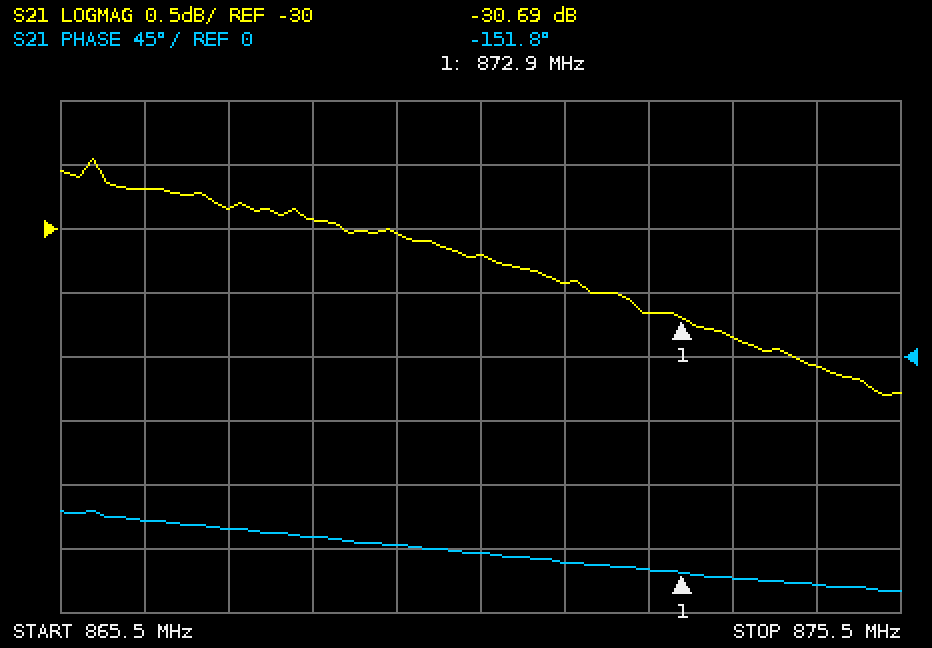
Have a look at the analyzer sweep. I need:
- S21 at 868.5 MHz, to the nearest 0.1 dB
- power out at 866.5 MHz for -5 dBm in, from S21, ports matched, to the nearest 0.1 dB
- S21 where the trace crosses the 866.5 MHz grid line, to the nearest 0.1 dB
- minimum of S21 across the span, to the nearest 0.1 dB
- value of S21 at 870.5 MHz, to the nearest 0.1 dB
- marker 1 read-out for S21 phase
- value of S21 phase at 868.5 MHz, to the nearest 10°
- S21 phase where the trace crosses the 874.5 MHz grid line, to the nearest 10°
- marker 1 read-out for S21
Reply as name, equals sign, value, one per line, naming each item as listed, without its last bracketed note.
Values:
S21 at 868.5 MHz, to the nearest 0.1 dB = -29.9 dB
power out at 866.5 MHz for -5 dBm in, from S21, ports matched, to the nearest 0.1 dB = -34.7 dBm
S21 where the trace crosses the 866.5 MHz grid line, to the nearest 0.1 dB = -29.7 dB
minimum of S21 across the span, to the nearest 0.1 dB = -31.3 dB
value of S21 at 870.5 MHz, to the nearest 0.1 dB = -30.2 dB
marker 1 read-out for S21 phase = -151.8°
value of S21 phase at 868.5 MHz, to the nearest 10° = -130°
S21 phase where the trace crosses the 874.5 MHz grid line, to the nearest 10° = -160°
marker 1 read-out for S21 = -30.69 dB
